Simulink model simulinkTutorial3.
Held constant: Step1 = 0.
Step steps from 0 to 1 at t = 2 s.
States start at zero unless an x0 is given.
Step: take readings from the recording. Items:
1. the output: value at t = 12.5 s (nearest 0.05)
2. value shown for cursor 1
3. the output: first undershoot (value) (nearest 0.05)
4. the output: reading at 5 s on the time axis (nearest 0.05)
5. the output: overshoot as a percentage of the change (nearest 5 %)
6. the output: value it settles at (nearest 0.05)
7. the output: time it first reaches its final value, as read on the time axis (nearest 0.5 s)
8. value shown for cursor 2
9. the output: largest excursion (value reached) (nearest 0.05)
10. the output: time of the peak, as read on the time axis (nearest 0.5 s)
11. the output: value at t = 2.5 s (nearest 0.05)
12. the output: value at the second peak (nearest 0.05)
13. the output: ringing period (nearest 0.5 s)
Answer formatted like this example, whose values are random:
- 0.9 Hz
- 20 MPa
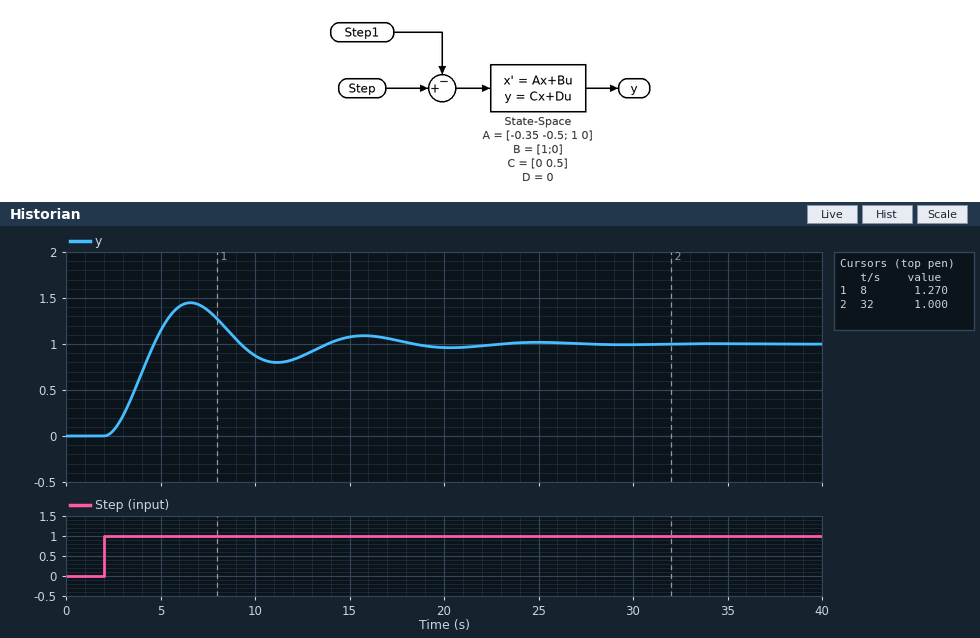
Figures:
- 0.85
- 1.270
- 0.80
- 1.15
- 45 %
- 1.00
- 4.5 s
- 1.000
- 1.45
- 6.5 s
- 0.05
- 1.10
- 9.0 s
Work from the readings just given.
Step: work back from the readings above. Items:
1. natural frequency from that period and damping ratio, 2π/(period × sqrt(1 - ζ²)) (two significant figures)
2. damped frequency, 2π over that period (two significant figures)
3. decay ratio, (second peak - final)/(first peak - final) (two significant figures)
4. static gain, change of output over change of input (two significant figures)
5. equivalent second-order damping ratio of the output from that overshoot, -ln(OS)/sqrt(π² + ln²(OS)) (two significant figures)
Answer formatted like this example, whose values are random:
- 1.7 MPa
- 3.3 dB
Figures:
- 0.72 rad/s
- 0.70 rad/s
- 0.22
- 1.0
- 0.25
